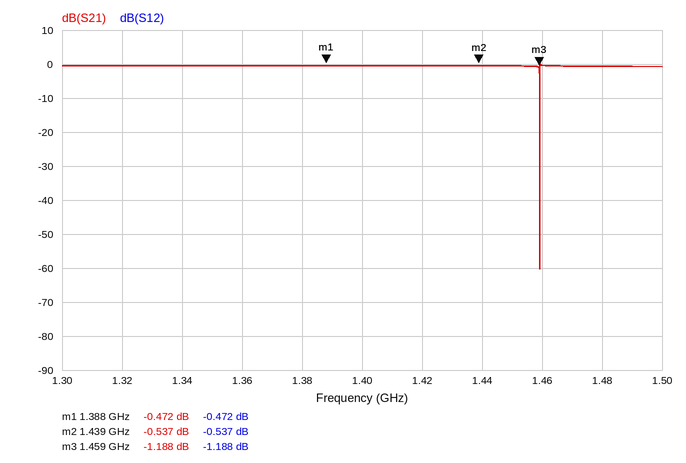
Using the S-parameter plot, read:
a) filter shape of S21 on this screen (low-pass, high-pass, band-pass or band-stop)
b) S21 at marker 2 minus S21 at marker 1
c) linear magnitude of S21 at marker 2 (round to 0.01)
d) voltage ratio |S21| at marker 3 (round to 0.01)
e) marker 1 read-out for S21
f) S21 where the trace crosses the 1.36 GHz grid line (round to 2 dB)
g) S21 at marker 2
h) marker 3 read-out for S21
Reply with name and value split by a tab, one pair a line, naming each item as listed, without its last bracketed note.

filter shape of S21 on this screen	band-stop
S21 at marker 2 minus S21 at marker 1	-0.065 dB
linear magnitude of S21 at marker 2	0.94
voltage ratio |S21| at marker 3	0.87
marker 1 read-out for S21	-0.472 dB
S21 where the trace crosses the 1.36 GHz grid line	0 dB
S21 at marker 2	-0.537 dB
marker 3 read-out for S21	-1.188 dB
